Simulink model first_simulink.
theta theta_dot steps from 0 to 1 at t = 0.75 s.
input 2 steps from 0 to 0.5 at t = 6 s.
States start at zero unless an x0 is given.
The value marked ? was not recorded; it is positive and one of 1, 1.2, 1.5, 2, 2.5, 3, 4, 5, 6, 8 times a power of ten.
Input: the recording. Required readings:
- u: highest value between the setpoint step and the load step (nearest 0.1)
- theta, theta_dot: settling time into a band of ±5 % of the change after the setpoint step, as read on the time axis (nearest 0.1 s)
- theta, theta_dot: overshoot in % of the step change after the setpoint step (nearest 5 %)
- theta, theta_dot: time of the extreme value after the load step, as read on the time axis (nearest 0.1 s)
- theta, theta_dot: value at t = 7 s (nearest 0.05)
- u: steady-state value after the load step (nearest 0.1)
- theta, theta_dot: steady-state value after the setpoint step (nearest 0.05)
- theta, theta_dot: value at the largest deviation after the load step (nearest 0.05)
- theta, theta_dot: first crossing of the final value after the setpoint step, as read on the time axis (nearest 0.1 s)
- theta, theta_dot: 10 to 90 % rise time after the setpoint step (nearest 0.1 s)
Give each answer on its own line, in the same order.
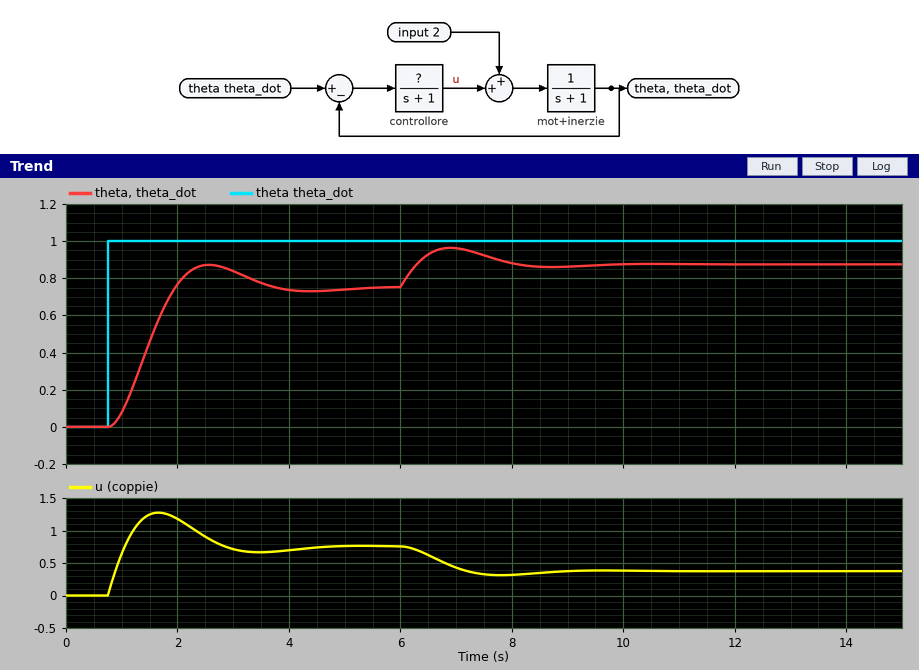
1.3
3.4 s
15 %
6.9 s
0.95
0.4
0.75
0.95
2.0 s
0.8 s
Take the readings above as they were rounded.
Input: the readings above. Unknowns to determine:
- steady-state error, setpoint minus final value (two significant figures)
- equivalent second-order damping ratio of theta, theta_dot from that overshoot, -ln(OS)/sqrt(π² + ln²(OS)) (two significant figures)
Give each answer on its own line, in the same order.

0.25
0.52
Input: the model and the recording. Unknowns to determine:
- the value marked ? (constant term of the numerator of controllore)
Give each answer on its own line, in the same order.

3
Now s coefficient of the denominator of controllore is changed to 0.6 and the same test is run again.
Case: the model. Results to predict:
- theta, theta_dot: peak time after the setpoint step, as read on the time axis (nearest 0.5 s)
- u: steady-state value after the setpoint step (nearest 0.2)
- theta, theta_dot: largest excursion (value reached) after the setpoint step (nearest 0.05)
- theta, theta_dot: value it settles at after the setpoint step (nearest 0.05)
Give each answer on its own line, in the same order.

2.0 s
0.8
0.85
0.75
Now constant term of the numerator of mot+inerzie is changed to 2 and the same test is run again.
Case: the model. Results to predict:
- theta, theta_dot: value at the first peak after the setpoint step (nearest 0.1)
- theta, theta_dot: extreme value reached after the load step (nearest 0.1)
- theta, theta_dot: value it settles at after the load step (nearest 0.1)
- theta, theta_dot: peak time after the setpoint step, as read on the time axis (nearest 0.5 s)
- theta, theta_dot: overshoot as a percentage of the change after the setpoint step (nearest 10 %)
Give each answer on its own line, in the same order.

1.1
1.2
1.0
2.0 s
30 %
